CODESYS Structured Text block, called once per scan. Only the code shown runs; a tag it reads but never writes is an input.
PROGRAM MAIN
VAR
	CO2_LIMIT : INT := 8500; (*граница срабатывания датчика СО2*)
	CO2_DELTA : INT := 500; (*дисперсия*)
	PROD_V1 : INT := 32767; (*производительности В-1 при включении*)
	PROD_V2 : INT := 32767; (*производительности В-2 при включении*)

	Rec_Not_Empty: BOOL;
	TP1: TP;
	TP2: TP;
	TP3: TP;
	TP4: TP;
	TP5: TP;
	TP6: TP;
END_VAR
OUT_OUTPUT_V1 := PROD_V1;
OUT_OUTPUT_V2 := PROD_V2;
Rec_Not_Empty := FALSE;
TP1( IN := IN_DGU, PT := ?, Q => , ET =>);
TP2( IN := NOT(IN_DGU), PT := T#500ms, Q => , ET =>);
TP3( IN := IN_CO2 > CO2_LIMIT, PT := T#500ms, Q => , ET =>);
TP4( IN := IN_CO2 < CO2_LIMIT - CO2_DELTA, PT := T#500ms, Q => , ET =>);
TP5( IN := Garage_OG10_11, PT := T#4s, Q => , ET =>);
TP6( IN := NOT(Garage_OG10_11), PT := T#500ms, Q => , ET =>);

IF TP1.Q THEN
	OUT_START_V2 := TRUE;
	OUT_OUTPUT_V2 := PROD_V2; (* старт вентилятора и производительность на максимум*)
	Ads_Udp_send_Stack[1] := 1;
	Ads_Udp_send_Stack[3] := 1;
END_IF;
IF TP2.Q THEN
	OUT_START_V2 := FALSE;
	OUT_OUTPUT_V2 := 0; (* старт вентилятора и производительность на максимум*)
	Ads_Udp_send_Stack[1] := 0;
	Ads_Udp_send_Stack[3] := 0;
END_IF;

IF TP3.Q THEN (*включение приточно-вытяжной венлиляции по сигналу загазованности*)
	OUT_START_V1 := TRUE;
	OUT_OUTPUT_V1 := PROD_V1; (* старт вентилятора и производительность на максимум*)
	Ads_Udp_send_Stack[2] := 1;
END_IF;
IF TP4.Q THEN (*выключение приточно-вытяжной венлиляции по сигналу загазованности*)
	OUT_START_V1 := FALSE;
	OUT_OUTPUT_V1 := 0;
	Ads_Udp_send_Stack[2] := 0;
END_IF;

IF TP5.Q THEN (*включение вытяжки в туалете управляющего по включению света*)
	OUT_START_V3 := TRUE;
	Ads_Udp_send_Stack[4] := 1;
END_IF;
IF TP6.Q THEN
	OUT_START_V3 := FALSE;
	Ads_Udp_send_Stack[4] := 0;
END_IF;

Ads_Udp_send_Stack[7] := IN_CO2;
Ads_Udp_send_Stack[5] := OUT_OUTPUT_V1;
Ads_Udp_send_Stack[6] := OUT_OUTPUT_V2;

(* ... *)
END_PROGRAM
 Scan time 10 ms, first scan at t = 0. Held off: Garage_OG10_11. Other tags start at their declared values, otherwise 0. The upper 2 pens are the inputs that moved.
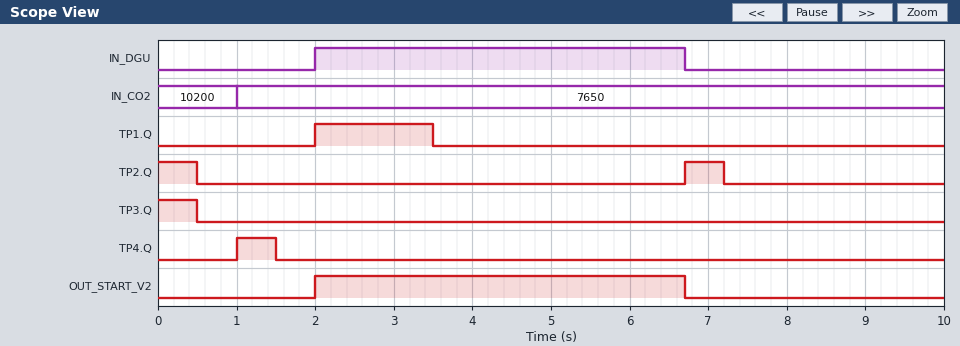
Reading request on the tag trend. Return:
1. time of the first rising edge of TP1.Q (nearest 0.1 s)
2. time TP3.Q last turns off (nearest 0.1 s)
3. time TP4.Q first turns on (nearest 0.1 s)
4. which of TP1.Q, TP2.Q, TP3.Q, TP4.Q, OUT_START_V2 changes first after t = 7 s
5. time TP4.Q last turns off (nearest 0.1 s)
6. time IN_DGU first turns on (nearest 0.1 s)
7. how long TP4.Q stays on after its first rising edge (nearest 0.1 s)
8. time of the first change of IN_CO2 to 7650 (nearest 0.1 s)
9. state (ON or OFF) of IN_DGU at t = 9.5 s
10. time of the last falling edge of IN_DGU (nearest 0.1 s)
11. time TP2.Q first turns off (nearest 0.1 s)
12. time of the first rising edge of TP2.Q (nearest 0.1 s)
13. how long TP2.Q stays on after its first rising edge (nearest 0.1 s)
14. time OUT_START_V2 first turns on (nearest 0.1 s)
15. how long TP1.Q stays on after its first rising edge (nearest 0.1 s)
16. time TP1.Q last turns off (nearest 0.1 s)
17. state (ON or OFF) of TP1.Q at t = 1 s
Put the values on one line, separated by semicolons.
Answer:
2.0 s; 0.5 s; 1.0 s; TP2.Q; 1.5 s; 2.0 s; 0.5 s; 1.0 s; OFF; 6.7 s; 0.5 s; 6.7 s; 0.5 s; 2.0 s; 1.5 s; 3.5 s; OFF
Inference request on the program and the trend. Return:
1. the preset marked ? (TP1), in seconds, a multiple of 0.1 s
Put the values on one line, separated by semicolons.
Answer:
1.5 s
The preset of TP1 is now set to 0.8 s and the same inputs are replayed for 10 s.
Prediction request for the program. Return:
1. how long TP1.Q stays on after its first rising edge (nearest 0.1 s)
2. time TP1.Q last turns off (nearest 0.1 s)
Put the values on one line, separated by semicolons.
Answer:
0.8 s; 2.8 s
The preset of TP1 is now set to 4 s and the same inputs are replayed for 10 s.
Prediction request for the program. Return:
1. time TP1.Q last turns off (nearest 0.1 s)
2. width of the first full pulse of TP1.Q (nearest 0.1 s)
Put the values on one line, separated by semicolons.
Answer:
6.0 s; 4.0 s
